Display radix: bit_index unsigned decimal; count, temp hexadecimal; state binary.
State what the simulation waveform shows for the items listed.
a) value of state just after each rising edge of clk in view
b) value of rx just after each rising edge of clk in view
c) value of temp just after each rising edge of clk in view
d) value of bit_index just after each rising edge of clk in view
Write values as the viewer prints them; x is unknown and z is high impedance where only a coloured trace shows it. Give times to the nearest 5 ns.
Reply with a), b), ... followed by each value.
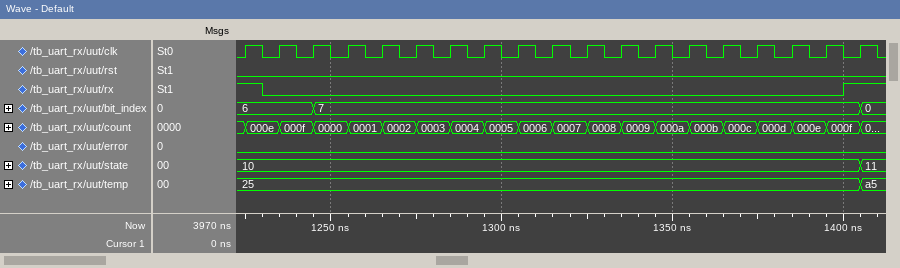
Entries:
a) 10, 10, 10, 10, 10, 10, 10, 10, 10, 10, 10, 10, 10, 10, 10, 10, 10, 10, 11
b) 1 0 0 0 0 0 0 0 0 0 0 0 0 0 0 0 0 0 1
c) 25, 25, 25, 25, 25, 25, 25, 25, 25, 25, 25, 25, 25, 25, 25, 25, 25, 25, a5
d) 6, 6, 7, 7, 7, 7, 7, 7, 7, 7, 7, 7, 7, 7, 7, 7, 7, 7, 0
